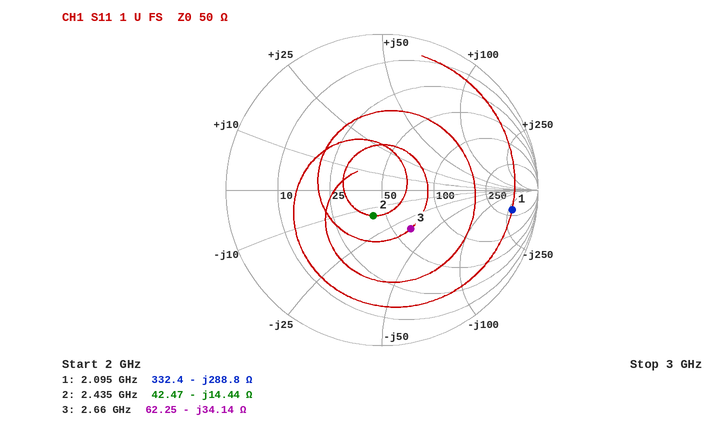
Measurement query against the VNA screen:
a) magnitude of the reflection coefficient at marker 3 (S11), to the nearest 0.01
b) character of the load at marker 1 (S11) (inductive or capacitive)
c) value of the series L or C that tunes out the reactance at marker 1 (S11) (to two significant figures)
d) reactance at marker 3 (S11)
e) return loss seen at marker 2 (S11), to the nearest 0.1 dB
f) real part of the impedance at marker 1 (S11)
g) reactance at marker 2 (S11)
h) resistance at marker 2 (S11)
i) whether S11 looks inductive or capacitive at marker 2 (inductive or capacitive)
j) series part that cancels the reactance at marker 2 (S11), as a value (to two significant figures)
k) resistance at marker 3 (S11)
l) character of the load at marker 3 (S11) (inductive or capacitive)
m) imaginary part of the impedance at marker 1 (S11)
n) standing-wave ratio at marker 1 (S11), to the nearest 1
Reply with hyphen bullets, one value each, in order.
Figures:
- 0.31
- capacitive
- 22 nH
- -34.14 Ω
- 15.2 dB
- 332.4 Ω
- -14.44 Ω
- 42.47 Ω
- capacitive
- 940 pH
- 62.25 Ω
- capacitive
- -288.8 Ω
- 12
